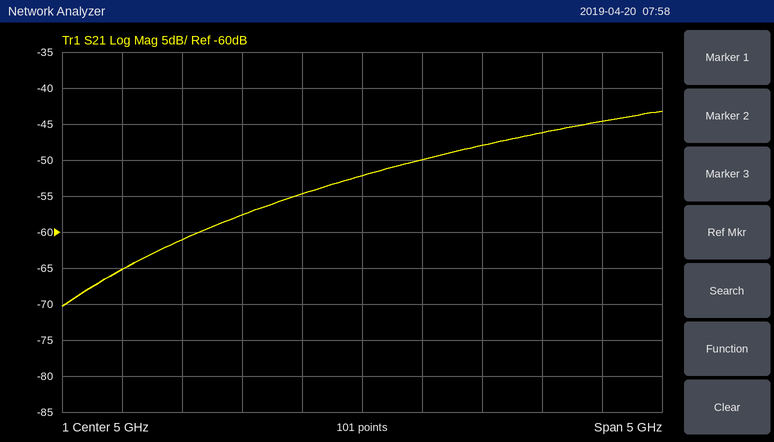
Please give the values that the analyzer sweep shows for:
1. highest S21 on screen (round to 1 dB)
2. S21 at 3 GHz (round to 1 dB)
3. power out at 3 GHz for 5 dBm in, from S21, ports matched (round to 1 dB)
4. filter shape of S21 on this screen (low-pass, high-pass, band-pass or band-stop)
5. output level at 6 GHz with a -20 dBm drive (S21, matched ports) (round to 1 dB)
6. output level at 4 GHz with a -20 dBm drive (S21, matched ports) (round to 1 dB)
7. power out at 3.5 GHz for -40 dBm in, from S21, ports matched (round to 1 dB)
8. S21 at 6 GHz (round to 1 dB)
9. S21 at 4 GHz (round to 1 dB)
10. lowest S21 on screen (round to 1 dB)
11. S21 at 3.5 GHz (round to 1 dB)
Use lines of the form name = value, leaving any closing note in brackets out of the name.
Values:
highest S21 on screen = -43 dB
S21 at 3 GHz = -65 dB
power out at 3 GHz for 5 dBm in, from S21, ports matched = -60 dBm
filter shape of S21 on this screen = high-pass
output level at 6 GHz with a -20 dBm drive (S21, matched ports) = -68 dBm
output level at 4 GHz with a -20 dBm drive (S21, matched ports) = -78 dBm
power out at 3.5 GHz for -40 dBm in, from S21, ports matched = -101 dBm
S21 at 6 GHz = -48 dB
S21 at 4 GHz = -58 dB
lowest S21 on screen = -70 dB
S21 at 3.5 GHz = -61 dB
